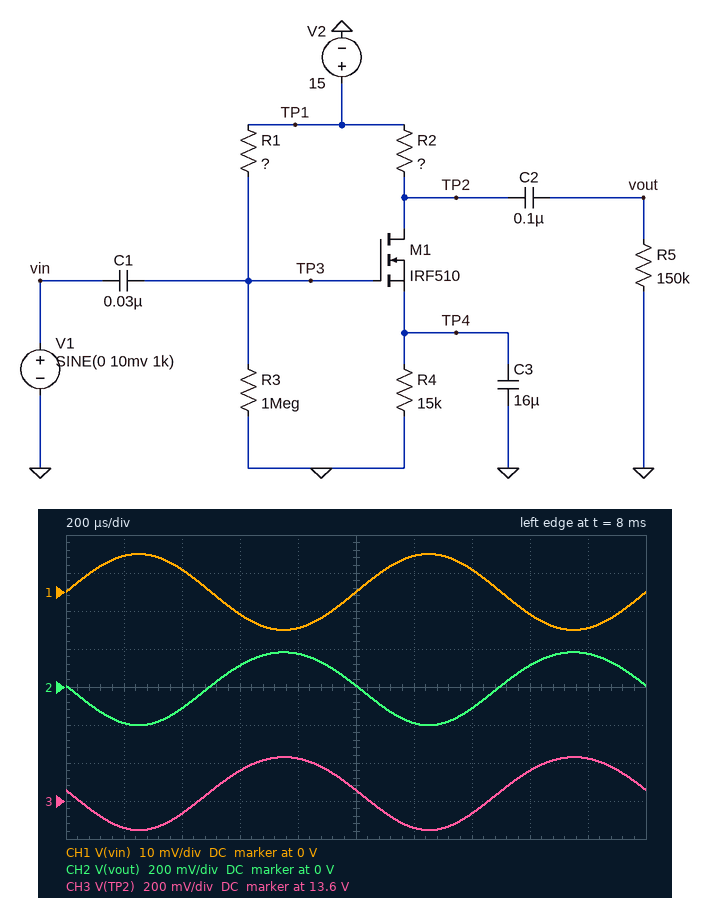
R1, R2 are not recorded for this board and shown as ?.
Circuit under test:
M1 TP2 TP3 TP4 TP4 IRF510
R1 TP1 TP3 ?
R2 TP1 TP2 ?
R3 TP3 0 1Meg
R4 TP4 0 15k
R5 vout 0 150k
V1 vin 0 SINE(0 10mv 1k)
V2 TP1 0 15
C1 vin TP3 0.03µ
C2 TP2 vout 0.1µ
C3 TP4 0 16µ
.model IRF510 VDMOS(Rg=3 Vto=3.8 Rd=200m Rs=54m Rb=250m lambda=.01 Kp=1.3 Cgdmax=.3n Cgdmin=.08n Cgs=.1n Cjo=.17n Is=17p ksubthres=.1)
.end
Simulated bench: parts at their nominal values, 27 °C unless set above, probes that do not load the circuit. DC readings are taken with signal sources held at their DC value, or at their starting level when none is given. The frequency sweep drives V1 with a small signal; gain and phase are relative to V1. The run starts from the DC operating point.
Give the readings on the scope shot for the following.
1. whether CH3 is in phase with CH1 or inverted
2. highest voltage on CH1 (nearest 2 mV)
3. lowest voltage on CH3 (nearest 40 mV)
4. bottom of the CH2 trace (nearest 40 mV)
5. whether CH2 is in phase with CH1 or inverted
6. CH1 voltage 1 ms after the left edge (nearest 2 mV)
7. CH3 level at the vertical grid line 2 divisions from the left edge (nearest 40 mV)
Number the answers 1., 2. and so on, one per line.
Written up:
1. inverted
2. 10 mV
3. 13.44 V
4. -200 mV
5. inverted
6. 0 V
7. 13.52 V
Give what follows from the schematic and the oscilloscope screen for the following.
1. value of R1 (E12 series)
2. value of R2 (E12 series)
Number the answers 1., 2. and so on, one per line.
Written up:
1. 2.7 MΩ
2. 39 kΩ
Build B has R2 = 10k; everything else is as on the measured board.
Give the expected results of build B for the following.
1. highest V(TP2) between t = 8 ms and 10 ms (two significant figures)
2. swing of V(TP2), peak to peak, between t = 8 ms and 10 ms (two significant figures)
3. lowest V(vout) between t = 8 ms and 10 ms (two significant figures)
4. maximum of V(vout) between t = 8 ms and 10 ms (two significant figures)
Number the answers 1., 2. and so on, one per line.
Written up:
1. 15 V
2. 120 mV
3. -64 mV
4. 58 mV
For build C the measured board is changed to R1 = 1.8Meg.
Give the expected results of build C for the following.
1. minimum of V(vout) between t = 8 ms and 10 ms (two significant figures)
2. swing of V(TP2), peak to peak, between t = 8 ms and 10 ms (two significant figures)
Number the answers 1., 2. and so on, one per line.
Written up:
1. -550 mV
2. 1.1 V
